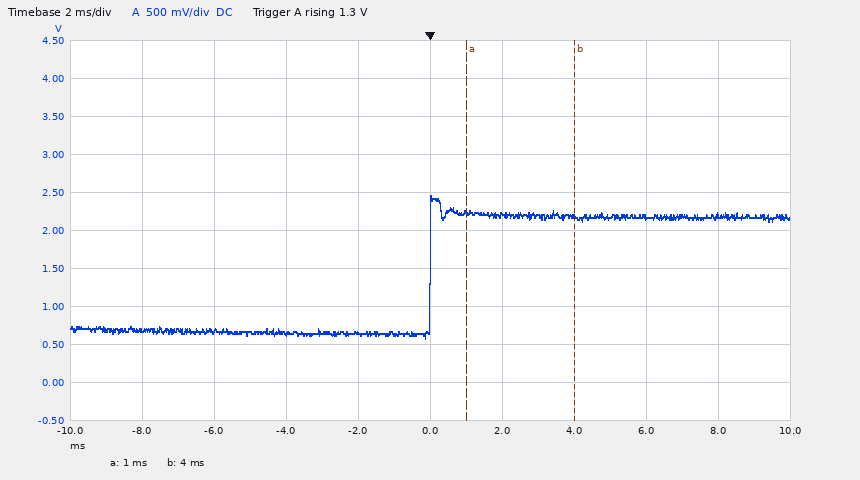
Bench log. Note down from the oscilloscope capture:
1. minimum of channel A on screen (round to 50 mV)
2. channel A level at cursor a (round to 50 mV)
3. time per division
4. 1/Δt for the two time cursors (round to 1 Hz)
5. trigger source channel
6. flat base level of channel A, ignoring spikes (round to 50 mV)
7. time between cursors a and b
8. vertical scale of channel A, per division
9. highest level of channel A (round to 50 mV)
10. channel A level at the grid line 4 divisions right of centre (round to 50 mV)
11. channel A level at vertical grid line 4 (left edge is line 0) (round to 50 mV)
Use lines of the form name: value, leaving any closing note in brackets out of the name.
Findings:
minimum of channel A on screen: 600 mV
channel A level at cursor a: 2.25 V
time per division: 2 ms
1/Δt for the two time cursors: 333 Hz
trigger source channel: channel A
flat base level of channel A, ignoring spikes: 650 mV
time between cursors a and b: 3.0 ms
vertical scale of channel A, per division: 500 mV
highest level of channel A: 2.45 V
channel A level at the grid line 4 divisions right of centre: 2.20 V
channel A level at vertical grid line 4 (left edge is line 0): 650 mV
